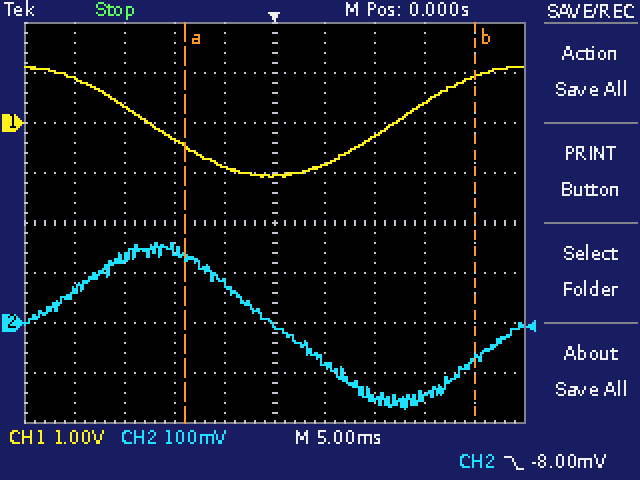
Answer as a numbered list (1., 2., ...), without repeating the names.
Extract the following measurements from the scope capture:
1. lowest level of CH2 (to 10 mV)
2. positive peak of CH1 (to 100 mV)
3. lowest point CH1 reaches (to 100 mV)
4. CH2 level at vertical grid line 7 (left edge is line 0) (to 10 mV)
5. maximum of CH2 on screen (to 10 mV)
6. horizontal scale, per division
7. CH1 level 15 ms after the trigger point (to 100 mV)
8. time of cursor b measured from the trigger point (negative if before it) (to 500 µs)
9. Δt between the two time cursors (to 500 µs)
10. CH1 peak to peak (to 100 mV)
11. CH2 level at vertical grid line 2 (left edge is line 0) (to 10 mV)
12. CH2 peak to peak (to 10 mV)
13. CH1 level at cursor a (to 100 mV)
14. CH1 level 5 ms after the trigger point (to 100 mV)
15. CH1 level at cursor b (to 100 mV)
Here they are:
1. -170 mV
2. 1.1 V
3. -1.1 V
4. -150 mV
5. 160 mV
6. 5 ms
7. 400 mV
8. +20.0 ms
9. 29.0 ms
10. 2.2 V
11. 130 mV
12. 330 mV
13. -500 mV
14. -800 mV
15. 900 mV
